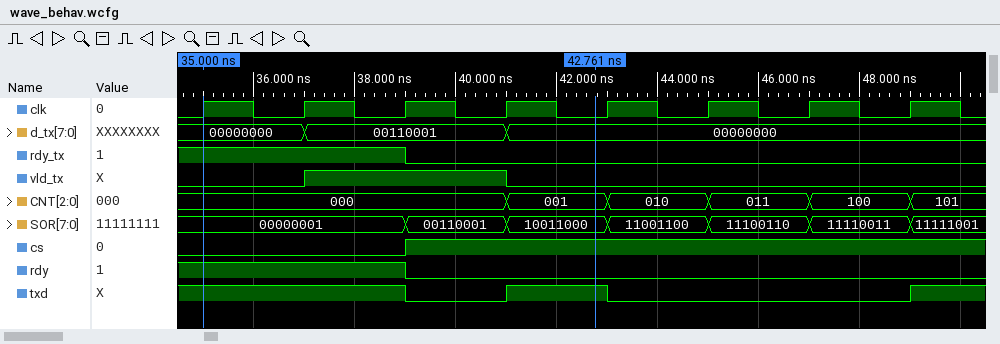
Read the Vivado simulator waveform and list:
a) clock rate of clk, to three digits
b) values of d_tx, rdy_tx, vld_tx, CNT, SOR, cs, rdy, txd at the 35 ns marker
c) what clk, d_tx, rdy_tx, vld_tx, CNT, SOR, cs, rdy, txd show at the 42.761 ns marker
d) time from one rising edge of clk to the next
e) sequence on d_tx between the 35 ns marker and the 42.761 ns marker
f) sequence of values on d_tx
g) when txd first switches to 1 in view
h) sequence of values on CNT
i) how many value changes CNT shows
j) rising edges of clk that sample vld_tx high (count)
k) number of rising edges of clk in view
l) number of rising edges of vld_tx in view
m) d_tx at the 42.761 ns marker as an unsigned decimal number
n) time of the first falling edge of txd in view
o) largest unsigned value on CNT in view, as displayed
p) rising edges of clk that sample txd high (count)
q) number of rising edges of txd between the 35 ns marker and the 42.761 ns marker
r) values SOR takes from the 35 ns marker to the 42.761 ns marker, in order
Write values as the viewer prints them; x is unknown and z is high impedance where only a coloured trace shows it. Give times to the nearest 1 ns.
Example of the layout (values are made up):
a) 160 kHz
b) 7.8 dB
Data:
a) 500 MHz
b) d_tx=00000000, rdy_tx=1, vld_tx=0, CNT=000, SOR=00000001, cs=0, rdy=1, txd=1
c) clk=0, d_tx=00000000, rdy_tx=0, vld_tx=0, CNT=001, SOR=10011000, cs=1, rdy=0, txd=1
d) 2 ns
e) 00000000, 00110001, 00000000
f) 00000000, 00110001, 00000000
g) 41 ns
h) 000, 001, 010, 011, 100, 101
i) 5
j) 2
k) 8
l) 1
m) 0
n) 39 ns
o) 101
p) 4
q) 1
r) 00000001, 00110001, 10011000
